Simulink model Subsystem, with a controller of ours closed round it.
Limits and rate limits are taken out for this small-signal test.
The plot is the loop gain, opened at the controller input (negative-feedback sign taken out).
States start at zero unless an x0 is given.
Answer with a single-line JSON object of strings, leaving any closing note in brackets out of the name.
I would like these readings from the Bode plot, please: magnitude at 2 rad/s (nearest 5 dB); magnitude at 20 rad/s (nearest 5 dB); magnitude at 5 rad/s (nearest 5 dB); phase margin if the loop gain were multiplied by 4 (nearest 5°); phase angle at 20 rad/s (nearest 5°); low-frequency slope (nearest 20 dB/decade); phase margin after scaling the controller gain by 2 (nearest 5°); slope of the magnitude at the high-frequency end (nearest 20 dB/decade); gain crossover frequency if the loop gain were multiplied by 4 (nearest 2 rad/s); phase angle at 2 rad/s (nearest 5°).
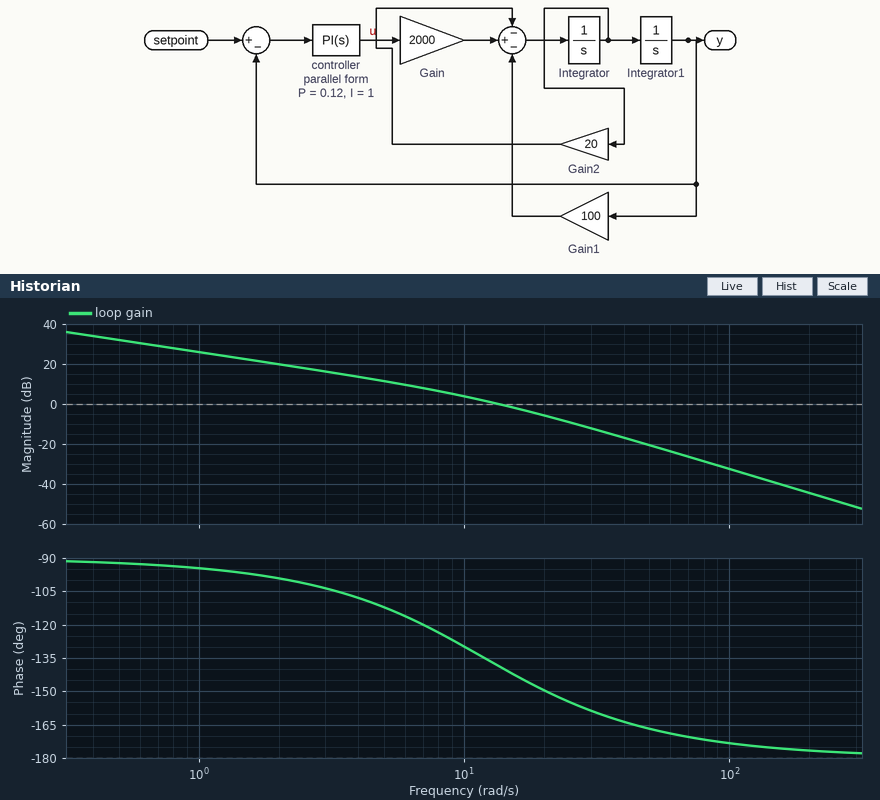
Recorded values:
{"magnitude at 2 rad/s": "20 dB", "magnitude at 20 rad/s": "-5 dB", "magnitude at 5 rad/s": "10 dB", "phase margin if the loop gain were multiplied by 4": "20°", "phase angle at 20 rad/s": "-150°", "low-frequency slope": "-20 dB/decade", "phase margin after scaling the controller gain by 2": "30°", "slope of the magnitude at the high-frequency end": "-40 dB/decade", "gain crossover frequency if the loop gain were multiplied by 4": "30 rad/s", "phase angle at 2 rad/s": "-100°"}
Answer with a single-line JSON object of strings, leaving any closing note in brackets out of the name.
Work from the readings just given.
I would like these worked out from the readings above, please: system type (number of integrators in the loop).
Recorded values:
{"system type": "1"}
